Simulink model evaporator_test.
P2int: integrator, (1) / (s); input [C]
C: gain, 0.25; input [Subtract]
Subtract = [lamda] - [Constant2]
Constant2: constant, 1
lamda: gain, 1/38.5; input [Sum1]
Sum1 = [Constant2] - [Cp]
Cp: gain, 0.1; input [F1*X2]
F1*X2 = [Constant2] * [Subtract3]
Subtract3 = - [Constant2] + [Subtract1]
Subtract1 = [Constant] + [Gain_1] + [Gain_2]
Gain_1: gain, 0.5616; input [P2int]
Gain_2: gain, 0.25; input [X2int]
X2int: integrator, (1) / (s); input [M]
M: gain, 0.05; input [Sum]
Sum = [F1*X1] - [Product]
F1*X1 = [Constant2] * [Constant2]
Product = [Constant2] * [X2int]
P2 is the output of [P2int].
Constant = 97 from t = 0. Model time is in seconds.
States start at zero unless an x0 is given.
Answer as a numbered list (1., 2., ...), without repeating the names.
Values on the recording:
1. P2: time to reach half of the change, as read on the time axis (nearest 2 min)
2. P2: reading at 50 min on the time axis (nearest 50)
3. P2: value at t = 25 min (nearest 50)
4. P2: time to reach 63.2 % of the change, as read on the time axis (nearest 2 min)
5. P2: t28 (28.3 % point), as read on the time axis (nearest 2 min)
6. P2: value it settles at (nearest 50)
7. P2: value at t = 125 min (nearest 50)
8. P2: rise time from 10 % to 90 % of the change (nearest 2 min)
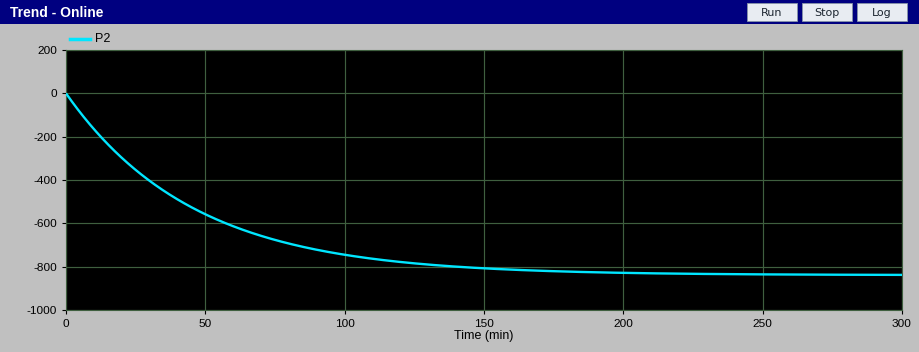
1. 32 min
2. -550
3. -350
4. 46 min
5. 16 min
6. -850
7. -800
8. 100 min
